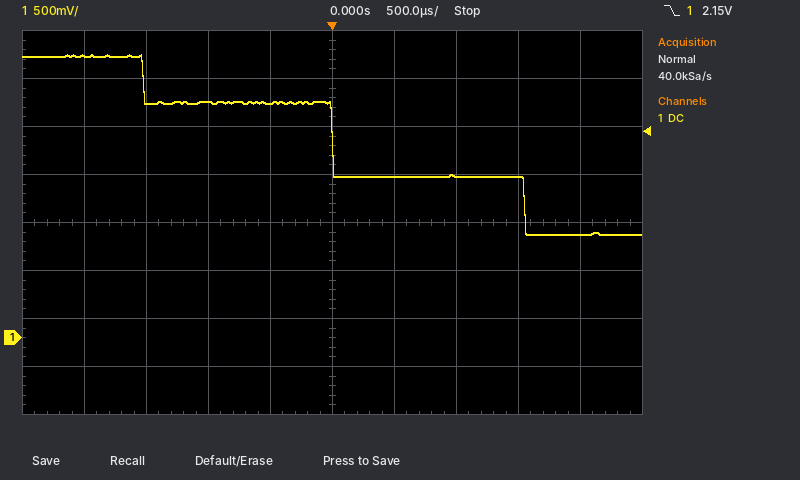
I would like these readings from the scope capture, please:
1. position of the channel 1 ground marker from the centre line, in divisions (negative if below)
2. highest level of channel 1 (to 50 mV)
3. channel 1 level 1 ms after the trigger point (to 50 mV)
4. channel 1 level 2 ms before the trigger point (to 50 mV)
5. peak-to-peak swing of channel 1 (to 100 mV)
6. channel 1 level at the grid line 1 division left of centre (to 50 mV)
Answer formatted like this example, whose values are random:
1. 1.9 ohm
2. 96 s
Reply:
1. -2.4 div
2. 2.95 V
3. 1.70 V
4. 2.95 V
5. 1.90 V
6. 2.45 V
